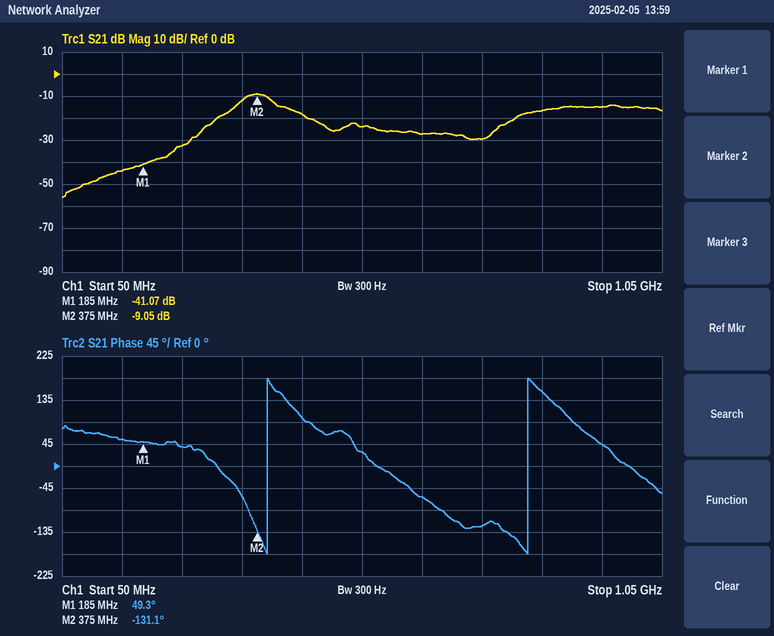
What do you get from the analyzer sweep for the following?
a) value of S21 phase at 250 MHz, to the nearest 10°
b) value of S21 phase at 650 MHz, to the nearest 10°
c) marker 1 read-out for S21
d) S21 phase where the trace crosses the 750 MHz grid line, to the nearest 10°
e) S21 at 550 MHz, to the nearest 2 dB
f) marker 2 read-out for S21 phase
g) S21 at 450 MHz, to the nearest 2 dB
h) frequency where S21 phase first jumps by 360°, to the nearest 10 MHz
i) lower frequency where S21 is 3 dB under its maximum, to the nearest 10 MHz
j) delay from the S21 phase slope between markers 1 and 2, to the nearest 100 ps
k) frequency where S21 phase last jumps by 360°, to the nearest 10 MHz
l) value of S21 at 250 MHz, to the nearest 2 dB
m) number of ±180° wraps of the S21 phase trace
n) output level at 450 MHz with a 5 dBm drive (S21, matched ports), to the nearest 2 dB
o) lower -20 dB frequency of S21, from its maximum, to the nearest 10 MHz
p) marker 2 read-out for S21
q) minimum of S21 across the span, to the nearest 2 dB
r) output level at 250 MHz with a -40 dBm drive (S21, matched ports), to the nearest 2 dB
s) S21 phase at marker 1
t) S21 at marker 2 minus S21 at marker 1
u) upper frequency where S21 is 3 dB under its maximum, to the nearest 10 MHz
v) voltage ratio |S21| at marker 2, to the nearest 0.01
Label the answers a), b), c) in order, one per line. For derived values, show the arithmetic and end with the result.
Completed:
a) 40°
b) -60°
c) -41.07 dB
d) -120°
e) -24 dB
f) -131.1°
g) -18 dB
h) 390 MHz
i) 350 MHz
j) −(-131.1° − (49.3°))/(360° × 190 MHz) ≈ 2.6 ns
k) 830 MHz
l) -32 dB
m) 2
n) 5 dBm + (-18 dB) = -14 dBm
o) 270 MHz
p) -9.05 dB
q) -56 dB
r) -40 dBm + (-32 dB) = -72 dBm
s) 49.3°
t) -9.05 − (-41.07) = 32.02 dB
u) 400 MHz
v) 10^(-9.05/20) ≈ 0.35
